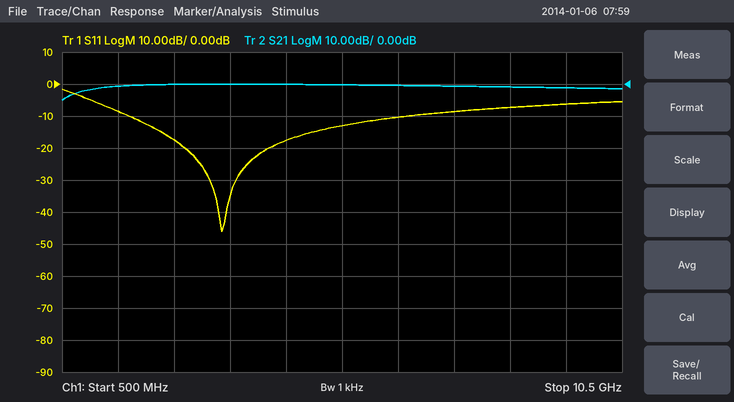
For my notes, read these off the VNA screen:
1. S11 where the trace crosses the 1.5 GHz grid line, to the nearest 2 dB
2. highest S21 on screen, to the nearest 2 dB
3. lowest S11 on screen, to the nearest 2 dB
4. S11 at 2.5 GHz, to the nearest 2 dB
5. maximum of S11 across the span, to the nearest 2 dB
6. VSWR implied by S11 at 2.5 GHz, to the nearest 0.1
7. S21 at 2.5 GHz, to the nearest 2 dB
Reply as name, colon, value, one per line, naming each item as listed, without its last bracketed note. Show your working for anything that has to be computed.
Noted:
S11 where the trace crosses the 1.5 GHz grid line, to the nearest 2 dB: -8 dB
highest S21 on screen, to the nearest 2 dB: 0 dB
lowest S11 on screen, to the nearest 2 dB: -46 dB
S11 at 2.5 GHz, to the nearest 2 dB: -18 dB
maximum of S11 across the span, to the nearest 2 dB: -2 dB
VSWR implied by S11 at 2.5 GHz, to the nearest 0.1: |Γ| = 10^(-18/20) = 0.1259; VSWR = (1 + 0.1259)/(1 − 0.1259) ≈ 1.3
S21 at 2.5 GHz, to the nearest 2 dB: 0 dB
